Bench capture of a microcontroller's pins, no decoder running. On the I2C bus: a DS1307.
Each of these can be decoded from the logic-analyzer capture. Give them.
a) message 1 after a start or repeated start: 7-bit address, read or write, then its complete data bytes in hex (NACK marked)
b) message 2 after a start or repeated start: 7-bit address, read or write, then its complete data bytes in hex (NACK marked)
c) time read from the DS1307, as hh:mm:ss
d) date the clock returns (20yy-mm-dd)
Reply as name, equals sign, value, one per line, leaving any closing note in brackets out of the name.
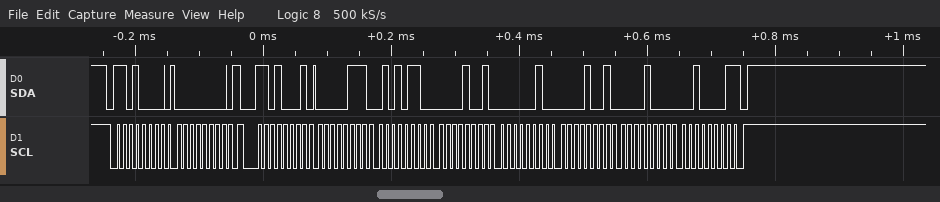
message 1 after a start or repeated start: 7-bit address, read or write, then its complete data bytes in hex = 0x68 write: 00
message 2 after a start or repeated start: 7-bit address, read or write, then its complete data bytes in hex = 0x68 read: 07 56 09 02 09 08 21 NACK
time read from the DS1307, as hh:mm:ss = 09:56:07
date the clock returns = 2021-08-09
